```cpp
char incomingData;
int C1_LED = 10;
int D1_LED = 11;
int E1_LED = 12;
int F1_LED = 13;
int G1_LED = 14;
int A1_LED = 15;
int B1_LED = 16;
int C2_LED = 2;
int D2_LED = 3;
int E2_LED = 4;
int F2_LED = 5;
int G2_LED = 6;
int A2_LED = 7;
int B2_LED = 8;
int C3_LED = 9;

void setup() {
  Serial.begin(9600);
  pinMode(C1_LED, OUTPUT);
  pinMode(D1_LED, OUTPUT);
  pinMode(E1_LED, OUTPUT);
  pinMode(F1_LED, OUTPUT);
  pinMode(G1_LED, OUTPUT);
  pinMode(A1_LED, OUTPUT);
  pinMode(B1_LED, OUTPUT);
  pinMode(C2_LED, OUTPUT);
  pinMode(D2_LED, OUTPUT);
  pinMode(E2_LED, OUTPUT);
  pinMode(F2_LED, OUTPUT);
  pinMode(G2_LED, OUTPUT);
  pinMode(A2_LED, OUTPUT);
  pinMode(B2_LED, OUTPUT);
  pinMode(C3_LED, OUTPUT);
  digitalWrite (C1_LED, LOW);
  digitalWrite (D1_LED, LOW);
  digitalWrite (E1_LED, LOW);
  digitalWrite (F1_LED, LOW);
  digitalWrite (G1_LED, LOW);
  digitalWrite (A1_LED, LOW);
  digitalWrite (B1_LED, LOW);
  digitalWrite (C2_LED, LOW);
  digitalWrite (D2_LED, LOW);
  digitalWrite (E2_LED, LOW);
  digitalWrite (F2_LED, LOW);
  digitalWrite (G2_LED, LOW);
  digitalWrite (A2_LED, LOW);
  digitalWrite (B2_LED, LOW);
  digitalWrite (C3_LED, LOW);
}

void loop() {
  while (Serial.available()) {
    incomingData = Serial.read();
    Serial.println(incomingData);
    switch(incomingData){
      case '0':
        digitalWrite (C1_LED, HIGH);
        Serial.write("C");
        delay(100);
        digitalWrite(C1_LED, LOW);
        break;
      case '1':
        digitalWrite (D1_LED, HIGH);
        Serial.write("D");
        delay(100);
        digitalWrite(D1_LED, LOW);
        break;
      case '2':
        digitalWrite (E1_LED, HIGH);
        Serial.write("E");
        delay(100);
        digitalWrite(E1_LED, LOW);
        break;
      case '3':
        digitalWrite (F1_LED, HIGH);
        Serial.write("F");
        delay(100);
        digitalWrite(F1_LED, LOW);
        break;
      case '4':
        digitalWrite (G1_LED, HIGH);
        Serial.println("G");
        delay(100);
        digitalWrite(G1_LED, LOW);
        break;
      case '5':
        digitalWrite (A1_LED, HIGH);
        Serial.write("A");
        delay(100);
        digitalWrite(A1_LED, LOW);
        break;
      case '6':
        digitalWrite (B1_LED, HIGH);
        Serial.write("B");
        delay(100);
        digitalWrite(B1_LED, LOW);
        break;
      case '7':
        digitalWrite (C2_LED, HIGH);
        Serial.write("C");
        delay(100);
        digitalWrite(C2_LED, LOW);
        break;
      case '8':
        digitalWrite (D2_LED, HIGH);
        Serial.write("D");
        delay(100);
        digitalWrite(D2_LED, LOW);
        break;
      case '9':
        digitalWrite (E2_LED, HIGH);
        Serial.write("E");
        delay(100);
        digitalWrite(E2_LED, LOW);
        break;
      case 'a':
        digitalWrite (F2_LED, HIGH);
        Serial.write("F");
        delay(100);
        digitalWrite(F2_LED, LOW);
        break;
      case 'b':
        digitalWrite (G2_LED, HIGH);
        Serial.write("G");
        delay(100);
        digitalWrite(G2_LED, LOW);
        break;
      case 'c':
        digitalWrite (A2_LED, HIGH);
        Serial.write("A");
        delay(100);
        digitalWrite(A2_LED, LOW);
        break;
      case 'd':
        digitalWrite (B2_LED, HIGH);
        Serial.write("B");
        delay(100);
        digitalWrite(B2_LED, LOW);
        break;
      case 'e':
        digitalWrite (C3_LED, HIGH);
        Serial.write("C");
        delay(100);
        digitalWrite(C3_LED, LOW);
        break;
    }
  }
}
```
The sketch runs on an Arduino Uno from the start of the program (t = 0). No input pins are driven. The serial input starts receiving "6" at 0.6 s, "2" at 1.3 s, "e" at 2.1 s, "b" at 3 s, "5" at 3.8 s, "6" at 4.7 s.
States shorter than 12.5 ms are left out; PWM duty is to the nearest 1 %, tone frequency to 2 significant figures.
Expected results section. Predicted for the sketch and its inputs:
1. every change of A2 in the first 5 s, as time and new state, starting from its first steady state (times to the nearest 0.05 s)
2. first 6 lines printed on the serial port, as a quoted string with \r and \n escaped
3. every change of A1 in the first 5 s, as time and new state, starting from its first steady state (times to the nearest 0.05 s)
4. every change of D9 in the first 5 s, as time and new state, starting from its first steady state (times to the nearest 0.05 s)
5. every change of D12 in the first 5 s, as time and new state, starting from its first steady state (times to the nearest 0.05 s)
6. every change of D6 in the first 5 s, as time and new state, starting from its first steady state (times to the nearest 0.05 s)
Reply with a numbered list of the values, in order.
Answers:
1. 0 s low; 0.6 s high; 0.7 s low; 4.7 s high; 4.8 s low
2. "6\r\nB2\r\nEe\r\nCb\r\nG5\r\nA6\r\n"
3. 0 s low; 3.8 s high; 3.9 s low
4. 0 s low; 2.1 s high; 2.2 s low
5. 0 s low; 1.3 s high; 1.4 s low
6. 0 s low; 3 s high; 3.1 s low
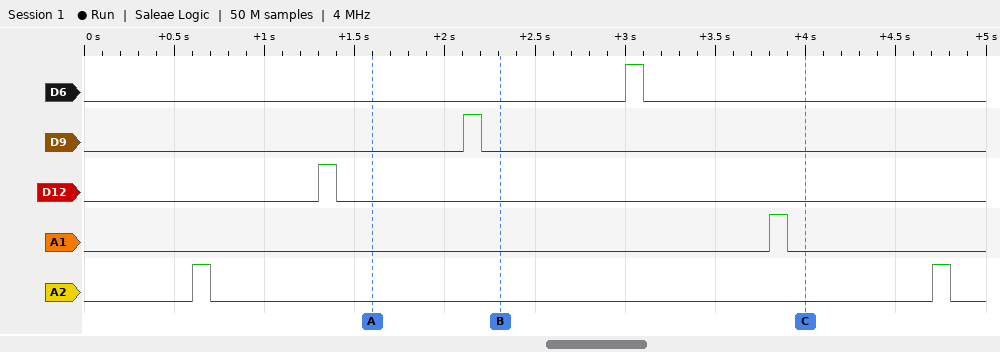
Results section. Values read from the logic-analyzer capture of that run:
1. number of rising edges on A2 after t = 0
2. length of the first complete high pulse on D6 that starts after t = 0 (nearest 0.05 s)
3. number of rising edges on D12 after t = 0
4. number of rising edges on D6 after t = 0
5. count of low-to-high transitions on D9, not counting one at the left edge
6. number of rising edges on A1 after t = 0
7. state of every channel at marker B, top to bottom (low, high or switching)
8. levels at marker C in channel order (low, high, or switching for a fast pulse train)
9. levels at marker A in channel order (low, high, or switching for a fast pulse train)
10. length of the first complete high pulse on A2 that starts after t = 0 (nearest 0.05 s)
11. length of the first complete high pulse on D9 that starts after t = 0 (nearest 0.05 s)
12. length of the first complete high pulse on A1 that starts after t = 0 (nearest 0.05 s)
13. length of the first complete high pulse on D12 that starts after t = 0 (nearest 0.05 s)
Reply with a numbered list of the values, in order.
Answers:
1. 2
2. 0.10 s
3. 1
4. 1
5. 1
6. 1
7. D6 low, D9 low, D12 low, A1 low, A2 low
8. D6 low, D9 low, D12 low, A1 low, A2 low
9. D6 low, D9 low, D12 low, A1 low, A2 low
10. 0.10 s
11. 0.10 s
12. 0.10 s
13. 0.10 s
